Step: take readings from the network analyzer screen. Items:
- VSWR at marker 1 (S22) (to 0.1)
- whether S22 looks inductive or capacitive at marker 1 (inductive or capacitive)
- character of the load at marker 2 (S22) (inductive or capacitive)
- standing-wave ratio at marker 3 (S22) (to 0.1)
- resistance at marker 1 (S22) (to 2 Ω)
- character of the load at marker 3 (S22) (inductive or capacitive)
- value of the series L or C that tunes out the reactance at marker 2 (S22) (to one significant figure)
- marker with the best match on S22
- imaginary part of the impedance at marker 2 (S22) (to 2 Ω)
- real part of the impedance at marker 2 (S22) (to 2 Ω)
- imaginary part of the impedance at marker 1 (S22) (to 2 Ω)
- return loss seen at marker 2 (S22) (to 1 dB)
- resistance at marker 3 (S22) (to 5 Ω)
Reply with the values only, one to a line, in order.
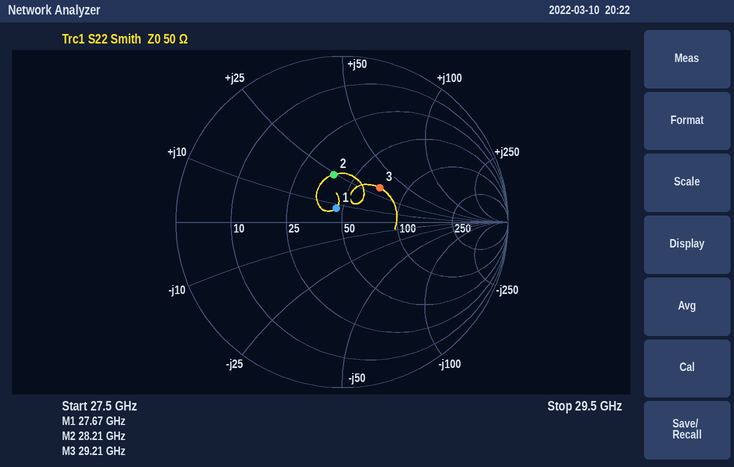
1.2
inductive
inductive
1.9
46 Ω
inductive
200 fF
marker 1
+24 Ω
38 Ω
+8 Ω
11 dB
70 Ω
